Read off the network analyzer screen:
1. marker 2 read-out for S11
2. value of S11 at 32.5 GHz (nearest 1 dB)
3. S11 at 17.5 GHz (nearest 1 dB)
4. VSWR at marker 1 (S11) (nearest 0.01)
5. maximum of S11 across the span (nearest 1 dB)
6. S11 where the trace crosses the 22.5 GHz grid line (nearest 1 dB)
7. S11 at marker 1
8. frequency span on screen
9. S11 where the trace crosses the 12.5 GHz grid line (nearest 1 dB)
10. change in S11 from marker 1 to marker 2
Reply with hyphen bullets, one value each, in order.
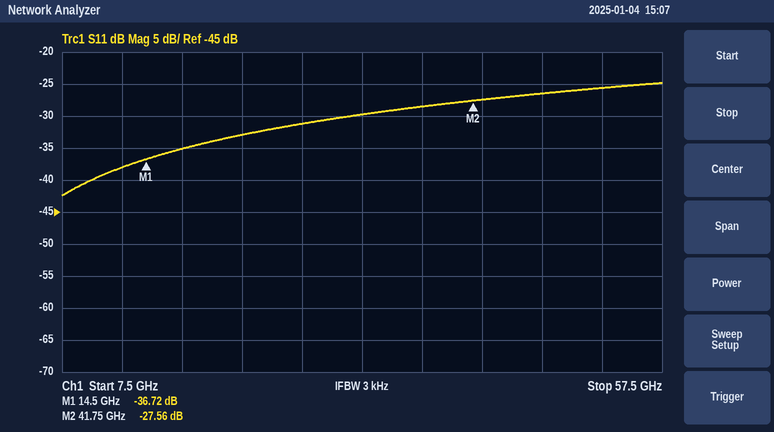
- -27.56 dB
- -30 dB
- -35 dB
- 1.03
- -25 dB
- -33 dB
- -36.72 dB
- 50 GHz
- -38 dB
- 9.16 dB
